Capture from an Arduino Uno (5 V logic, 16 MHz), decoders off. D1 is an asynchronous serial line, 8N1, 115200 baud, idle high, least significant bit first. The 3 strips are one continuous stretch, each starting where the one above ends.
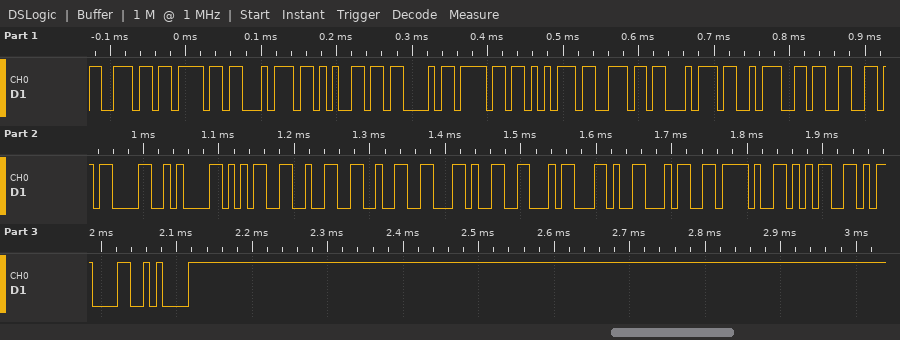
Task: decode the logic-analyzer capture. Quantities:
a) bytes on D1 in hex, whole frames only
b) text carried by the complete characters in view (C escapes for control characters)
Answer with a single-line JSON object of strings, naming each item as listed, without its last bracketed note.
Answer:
{"bytes on D1 in hex, whole frames only": "6E 6F 74 65 43 6F 75 6E 74 3A 33 0D 0A 35 32 32 2C 46 2C 34 2F 35 0D 0A", "text carried by the complete characters in view": "\"noteCount:3\\r\\n522,F,4/5\\r\\n\""}
